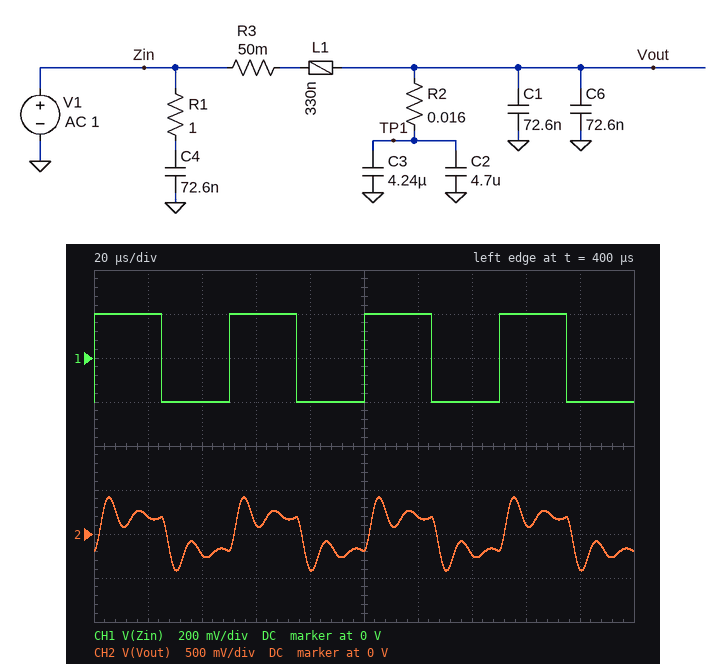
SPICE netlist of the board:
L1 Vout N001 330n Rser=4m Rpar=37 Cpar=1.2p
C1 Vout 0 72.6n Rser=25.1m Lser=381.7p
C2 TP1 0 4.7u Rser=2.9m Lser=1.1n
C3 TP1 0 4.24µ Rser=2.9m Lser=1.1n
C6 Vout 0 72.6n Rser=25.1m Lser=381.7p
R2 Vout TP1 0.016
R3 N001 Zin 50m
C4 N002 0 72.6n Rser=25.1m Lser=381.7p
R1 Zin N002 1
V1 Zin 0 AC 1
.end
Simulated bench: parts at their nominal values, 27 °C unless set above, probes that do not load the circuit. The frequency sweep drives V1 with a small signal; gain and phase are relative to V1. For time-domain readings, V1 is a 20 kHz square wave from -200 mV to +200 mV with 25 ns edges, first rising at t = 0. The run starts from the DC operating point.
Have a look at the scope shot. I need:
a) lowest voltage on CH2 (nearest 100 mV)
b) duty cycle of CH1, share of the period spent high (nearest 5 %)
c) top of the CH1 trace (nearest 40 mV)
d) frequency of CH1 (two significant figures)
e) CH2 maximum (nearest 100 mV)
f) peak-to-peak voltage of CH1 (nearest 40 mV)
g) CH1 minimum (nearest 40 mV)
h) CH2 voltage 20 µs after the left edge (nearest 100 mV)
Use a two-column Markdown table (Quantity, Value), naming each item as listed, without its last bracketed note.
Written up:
| Quantity | Value |
|---|---|
| lowest voltage on CH2 | -400 mV |
| duty cycle of CH1, share of the period spent high | 50 % |
| top of the CH1 trace | 200 mV |
| frequency of CH1 | 20 kHz |
| CH2 maximum | 400 mV |
| peak-to-peak voltage of CH1 | 400 mV |
| CH1 minimum | -200 mV |
| CH2 voltage 20 µs after the left edge | 200 mV |
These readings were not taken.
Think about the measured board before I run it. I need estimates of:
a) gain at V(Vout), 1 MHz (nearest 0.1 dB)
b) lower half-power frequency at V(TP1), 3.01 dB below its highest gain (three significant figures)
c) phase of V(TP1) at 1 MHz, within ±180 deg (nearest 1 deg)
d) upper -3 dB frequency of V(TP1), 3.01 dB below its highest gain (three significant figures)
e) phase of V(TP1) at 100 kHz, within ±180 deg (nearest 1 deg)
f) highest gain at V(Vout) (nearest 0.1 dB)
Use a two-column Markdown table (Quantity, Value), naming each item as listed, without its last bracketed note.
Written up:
| Quantity | Value |
|---|---|
| gain at V(Vout), 1 MHz | -39.3 dB |
| lower half-power frequency at V(TP1), 3.01 dB below its highest gain | 68.6 kHz |
| phase of V(TP1) at 1 MHz, within ±180 deg | -170 deg |
| upper -3 dB frequency of V(TP1), 3.01 dB below its highest gain | 105 kHz |
| phase of V(TP1) at 100 kHz, within ±180 deg | -114 deg |
| highest gain at V(Vout) | 8.7 dB |
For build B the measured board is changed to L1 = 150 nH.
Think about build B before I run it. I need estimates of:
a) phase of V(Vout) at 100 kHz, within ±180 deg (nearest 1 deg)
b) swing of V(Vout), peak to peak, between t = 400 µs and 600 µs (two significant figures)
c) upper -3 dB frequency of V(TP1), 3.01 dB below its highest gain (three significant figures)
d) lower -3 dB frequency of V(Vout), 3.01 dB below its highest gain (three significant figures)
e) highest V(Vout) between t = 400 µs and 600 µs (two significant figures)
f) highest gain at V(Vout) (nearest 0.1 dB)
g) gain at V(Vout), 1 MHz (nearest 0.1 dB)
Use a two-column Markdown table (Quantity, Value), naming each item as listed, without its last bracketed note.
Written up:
| Quantity | Value |
|---|---|
| phase of V(Vout) at 100 kHz, within ±180 deg | -36 deg |
| swing of V(Vout), peak to peak, between t = 400 µs and 600 µs | 730 mV |
| upper -3 dB frequency of V(TP1), 3.01 dB below its highest gain | 160 kHz |
| lower -3 dB frequency of V(Vout), 3.01 dB below its highest gain | 76.6 kHz |
| highest V(Vout) between t = 400 µs and 600 µs | 360 mV |
| highest gain at V(Vout) | 5.5 dB |
| gain at V(Vout), 1 MHz | -32.4 dB |
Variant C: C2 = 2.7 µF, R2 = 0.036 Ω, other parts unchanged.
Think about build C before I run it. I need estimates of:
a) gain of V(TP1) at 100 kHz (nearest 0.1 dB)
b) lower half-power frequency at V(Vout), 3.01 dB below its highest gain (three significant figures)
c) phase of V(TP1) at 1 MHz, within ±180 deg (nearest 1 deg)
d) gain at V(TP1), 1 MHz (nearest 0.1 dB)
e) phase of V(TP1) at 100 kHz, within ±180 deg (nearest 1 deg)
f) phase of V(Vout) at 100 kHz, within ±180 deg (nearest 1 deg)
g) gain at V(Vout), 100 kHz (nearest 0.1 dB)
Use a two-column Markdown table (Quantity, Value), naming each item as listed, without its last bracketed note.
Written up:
| Quantity | Value |
|---|---|
| gain of V(TP1) at 100 kHz | 7.7 dB |
| lower half-power frequency at V(Vout), 3.01 dB below its highest gain | 73.7 kHz |
| phase of V(TP1) at 1 MHz, within ±180 deg | -172 deg |
| gain at V(TP1), 1 MHz | -40.7 dB |
| phase of V(TP1) at 100 kHz, within ±180 deg | -79 deg |
| phase of V(Vout) at 100 kHz, within ±180 deg | -70 deg |
| gain at V(Vout), 100 kHz | 7.8 dB |
